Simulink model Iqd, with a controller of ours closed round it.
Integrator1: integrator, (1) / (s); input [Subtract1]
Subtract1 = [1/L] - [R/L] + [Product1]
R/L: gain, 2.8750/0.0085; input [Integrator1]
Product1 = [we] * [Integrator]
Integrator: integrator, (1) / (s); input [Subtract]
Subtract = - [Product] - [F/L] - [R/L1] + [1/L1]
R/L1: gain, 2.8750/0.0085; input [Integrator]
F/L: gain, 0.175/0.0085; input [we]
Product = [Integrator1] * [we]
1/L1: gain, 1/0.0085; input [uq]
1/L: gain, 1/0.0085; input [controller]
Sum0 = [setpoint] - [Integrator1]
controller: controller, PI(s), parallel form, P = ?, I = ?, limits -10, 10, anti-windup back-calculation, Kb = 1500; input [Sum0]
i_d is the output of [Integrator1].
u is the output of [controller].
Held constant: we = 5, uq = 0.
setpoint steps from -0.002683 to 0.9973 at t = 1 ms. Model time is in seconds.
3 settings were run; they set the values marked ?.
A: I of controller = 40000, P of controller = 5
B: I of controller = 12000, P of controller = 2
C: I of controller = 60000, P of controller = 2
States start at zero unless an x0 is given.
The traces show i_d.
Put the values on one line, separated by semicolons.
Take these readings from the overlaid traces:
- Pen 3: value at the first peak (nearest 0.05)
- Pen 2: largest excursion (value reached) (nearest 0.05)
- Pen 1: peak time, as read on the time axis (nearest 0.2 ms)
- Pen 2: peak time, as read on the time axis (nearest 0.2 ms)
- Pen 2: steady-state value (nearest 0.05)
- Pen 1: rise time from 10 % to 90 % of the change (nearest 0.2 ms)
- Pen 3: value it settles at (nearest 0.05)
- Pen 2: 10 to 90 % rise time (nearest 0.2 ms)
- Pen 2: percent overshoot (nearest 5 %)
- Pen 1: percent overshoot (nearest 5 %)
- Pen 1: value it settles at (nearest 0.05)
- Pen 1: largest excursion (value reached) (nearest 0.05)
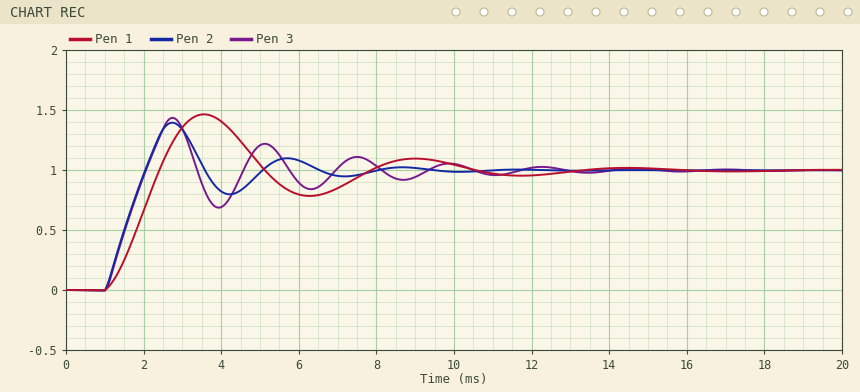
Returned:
1.45; 1.40; 3.6 ms; 2.8 ms; 1.00; 1.0 ms; 1.00; 0.8 ms; 40 %; 45 %; 1.00; 1.45
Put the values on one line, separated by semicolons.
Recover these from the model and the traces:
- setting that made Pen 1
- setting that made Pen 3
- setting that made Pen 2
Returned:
B; C; A
